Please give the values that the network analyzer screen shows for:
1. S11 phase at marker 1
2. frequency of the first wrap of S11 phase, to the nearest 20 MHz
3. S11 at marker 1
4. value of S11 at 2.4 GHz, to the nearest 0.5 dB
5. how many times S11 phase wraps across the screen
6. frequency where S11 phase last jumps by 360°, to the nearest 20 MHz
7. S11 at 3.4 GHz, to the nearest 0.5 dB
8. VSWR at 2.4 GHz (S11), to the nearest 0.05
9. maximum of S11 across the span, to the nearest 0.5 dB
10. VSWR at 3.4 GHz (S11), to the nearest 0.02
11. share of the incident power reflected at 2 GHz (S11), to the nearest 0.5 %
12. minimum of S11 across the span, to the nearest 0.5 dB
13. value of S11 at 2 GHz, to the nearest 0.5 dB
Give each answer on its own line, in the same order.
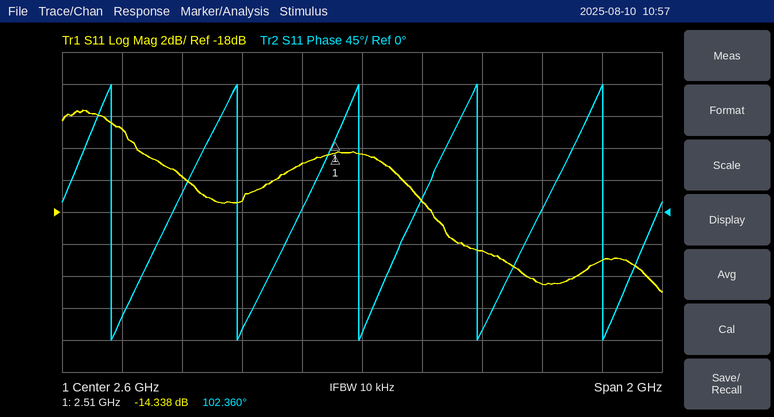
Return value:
102.360°
1.76 GHz
-14.338 dB
-15.0 dB
5
3.40 GHz
-21.0 dB
1.45
-11.5 dB
1.20
2.5 %
-23.0 dB
-16.0 dB
